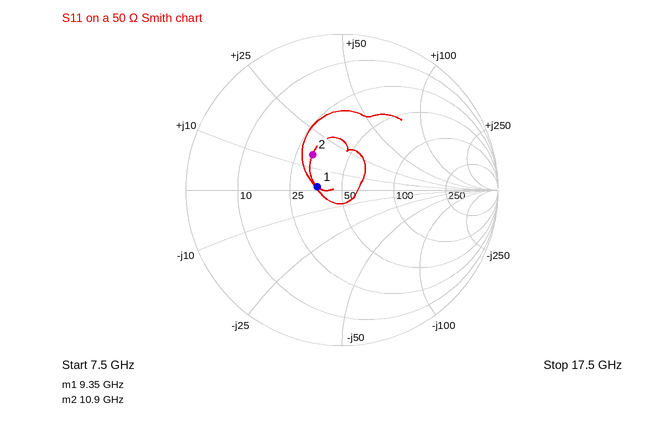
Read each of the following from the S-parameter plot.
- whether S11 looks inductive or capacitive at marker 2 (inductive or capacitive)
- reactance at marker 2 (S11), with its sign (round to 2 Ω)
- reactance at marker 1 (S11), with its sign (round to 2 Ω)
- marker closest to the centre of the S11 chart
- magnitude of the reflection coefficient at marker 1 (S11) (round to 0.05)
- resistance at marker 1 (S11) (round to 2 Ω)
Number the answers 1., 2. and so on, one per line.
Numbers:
1. inductive
2. +16 Ω
3. +2 Ω
4. marker 1
5. 0.15
6. 36 Ω
